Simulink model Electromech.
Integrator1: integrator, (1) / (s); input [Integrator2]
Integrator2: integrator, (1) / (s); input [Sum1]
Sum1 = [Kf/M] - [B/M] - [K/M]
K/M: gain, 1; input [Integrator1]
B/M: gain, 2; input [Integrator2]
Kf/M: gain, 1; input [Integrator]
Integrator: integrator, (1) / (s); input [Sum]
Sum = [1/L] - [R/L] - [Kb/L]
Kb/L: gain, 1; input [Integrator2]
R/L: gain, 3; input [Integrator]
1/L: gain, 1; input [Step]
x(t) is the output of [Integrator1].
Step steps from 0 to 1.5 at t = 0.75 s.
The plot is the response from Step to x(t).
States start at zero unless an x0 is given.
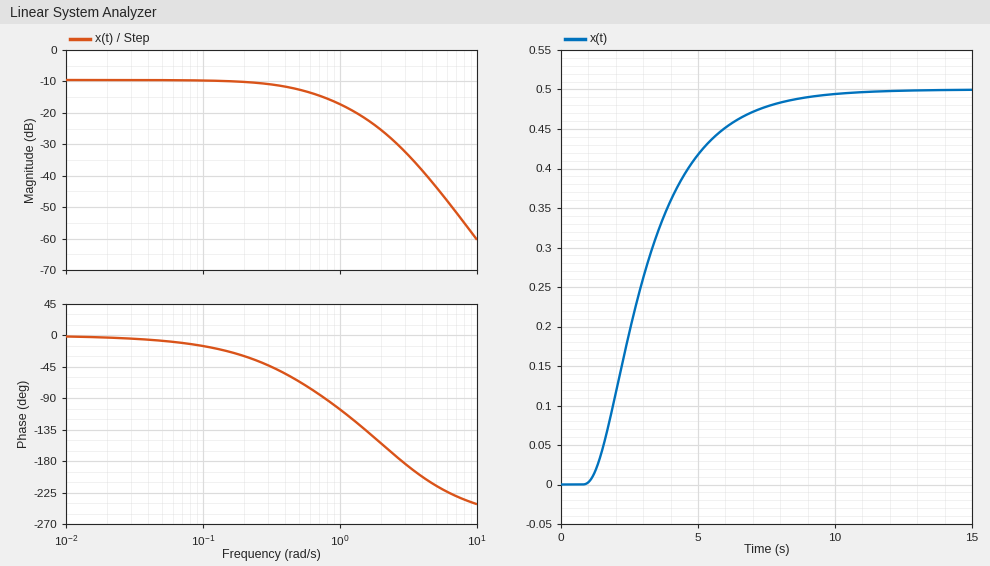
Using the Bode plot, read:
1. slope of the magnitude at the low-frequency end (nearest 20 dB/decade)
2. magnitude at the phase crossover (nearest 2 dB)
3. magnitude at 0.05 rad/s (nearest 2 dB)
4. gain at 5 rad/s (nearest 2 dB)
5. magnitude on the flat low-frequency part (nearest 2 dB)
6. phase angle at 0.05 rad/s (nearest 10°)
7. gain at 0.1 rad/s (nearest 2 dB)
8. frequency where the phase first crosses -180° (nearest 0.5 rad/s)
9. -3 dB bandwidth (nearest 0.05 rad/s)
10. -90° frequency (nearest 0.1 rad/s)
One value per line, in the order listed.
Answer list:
0 dB/decade
-32 dB
-10 dB
-44 dB
-10 dB
-10°
-10 dB
3.0 rad/s
0.50 rad/s
0.8 rad/s
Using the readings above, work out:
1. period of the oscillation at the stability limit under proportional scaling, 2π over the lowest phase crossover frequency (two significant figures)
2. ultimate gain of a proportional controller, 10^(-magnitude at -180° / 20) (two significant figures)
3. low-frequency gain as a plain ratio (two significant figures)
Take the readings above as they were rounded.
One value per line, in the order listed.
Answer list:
2.1 s
40
0.32
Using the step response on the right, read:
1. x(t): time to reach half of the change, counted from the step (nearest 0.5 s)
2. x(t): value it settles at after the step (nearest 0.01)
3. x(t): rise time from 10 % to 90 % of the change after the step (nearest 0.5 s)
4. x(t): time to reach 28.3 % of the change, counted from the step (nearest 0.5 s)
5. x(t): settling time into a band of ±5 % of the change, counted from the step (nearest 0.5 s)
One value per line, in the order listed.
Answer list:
2.0 s
0.50
4.5 s
1.5 s
6.5 s
